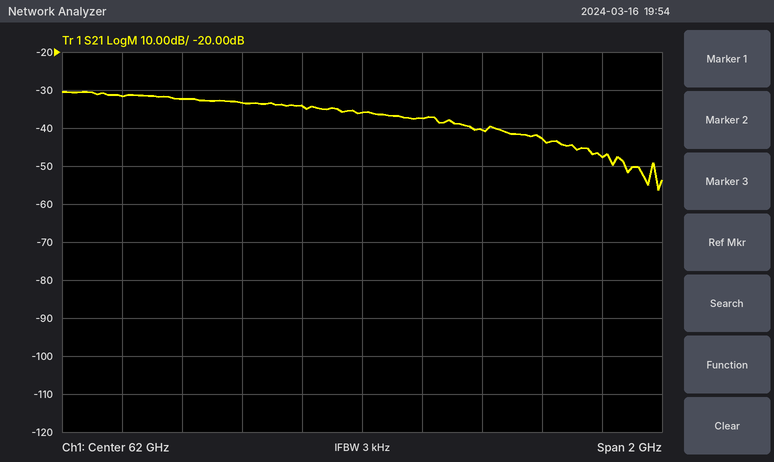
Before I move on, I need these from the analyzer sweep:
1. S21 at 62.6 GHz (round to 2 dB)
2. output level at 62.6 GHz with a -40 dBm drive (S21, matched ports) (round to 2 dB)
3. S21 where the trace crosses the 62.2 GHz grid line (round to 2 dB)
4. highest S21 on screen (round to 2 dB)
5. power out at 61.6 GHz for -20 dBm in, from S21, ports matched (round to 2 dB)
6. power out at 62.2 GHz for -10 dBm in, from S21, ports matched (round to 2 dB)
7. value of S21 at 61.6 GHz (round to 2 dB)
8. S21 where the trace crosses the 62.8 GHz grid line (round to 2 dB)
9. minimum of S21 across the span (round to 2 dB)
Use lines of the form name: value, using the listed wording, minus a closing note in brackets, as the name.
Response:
S21 at 62.6 GHz: -42 dB
output level at 62.6 GHz with a -40 dBm drive (S21, matched ports): -82 dBm
S21 where the trace crosses the 62.2 GHz grid line: -38 dB
highest S21 on screen: -30 dB
power out at 61.6 GHz for -20 dBm in, from S21, ports matched: -54 dBm
power out at 62.2 GHz for -10 dBm in, from S21, ports matched: -48 dBm
value of S21 at 61.6 GHz: -34 dB
S21 where the trace crosses the 62.8 GHz grid line: -48 dB
minimum of S21 across the span: -56 dB
